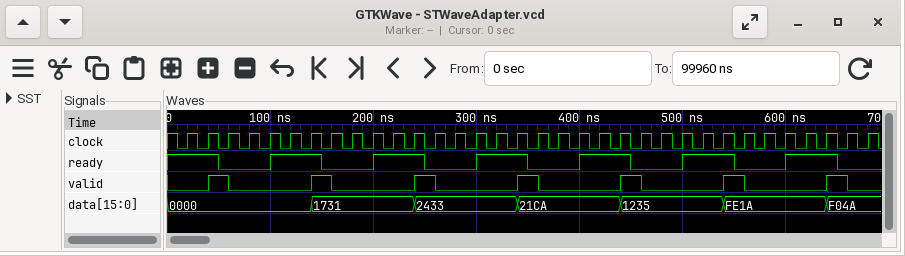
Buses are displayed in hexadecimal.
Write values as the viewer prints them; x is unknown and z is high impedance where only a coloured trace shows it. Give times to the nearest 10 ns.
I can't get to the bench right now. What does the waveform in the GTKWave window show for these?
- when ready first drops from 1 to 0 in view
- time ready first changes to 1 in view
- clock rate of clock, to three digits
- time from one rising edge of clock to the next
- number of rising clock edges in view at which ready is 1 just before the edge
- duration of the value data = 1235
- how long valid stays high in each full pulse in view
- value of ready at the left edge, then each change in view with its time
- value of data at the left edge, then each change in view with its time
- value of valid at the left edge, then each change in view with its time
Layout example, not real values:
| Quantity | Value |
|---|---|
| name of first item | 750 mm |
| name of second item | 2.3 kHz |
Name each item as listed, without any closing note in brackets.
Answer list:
| Quantity | Value |
|---|---|
| when ready first drops from 1 to 0 in view | 50 ns |
| time ready first changes to 1 in view | 100 ns |
| clock rate of clock, to three digits | 50.0 MHz |
| time from one rising edge of clock to the next | 20 ns |
| number of rising clock edges in view at which ready is 1 just before the edge | 14 |
| duration of the value data = 1235 | 100 ns |
| how long valid stays high in each full pulse in view | 20 ns, 20 ns, 20 ns, 20 ns, 20 ns, 20 ns, 20 ns |
| value of ready at the left edge, then each change in view with its time | 1, 0 at 50 ns, 1 at 100 ns, 0 at 150 ns, 1 at 200 ns, 0 at 250 ns, 1 at 300 ns, 0 at 350 ns, 1 at 400 ns, 0 at 450 ns, 1 at 500 ns, 0 at 550 ns, 1 at 600 ns, 0 at 650 ns |
| value of data at the left edge, then each change in view with its time | 0000, 1731 at 140 ns, 2433 at 240 ns, 21CA at 340 ns, 1235 at 440 ns, FE1A at 540 ns, F04A at 640 ns |
| value of valid at the left edge, then each change in view with its time | 0, 1 at 40 ns, 0 at 60 ns, 1 at 140 ns, 0 at 160 ns, 1 at 240 ns, 0 at 260 ns, 1 at 340 ns, 0 at 360 ns, 1 at 440 ns, 0 at 460 ns, 1 at 540 ns, 0 at 560 ns, 1 at 640 ns, 0 at 660 ns |
